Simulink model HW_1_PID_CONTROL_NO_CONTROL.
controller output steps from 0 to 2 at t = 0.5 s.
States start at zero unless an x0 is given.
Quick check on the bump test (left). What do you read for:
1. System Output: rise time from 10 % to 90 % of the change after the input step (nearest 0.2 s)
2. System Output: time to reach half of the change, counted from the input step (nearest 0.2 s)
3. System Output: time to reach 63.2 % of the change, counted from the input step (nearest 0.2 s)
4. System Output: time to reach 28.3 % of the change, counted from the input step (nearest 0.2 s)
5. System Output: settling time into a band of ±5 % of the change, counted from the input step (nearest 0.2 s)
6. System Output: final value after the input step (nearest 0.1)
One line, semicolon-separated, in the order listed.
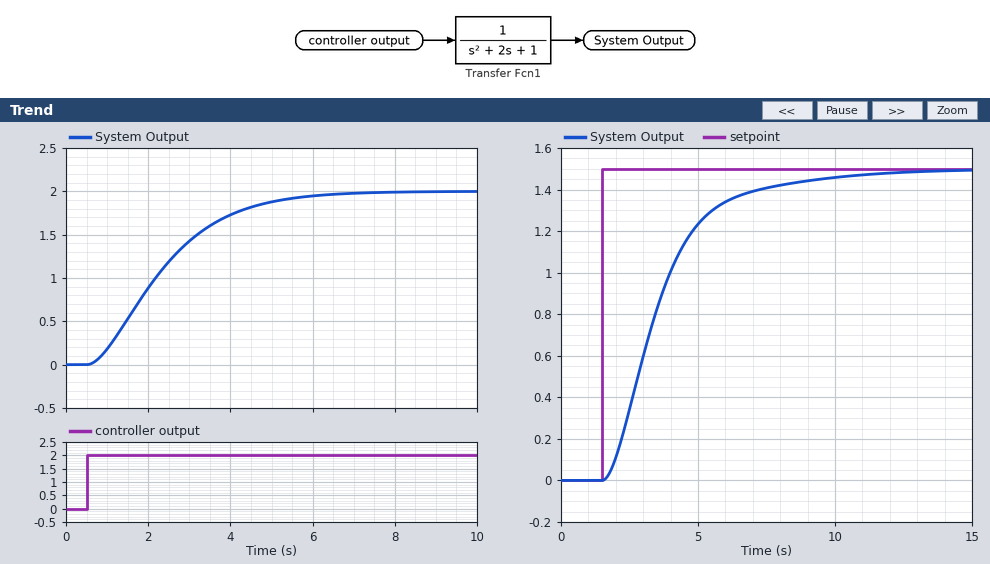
3.4 s; 1.6 s; 2.2 s; 1.0 s; 4.8 s; 2.0
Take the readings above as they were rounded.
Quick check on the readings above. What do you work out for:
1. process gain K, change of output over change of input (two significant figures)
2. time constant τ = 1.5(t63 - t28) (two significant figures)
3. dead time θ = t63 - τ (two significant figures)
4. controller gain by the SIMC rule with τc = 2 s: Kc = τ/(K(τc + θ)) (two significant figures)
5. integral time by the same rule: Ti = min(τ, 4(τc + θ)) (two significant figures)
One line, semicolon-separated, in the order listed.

1.0; 1.8 s; 0.40 s; 0.75; 1.8 s
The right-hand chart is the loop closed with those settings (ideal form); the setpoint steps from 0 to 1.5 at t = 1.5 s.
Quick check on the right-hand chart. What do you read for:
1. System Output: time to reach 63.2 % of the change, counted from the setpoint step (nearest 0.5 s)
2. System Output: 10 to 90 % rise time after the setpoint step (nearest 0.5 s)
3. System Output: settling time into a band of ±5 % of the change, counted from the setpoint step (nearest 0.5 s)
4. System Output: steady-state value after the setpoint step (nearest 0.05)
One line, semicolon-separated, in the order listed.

2.5 s; 4.0 s; 6.5 s; 1.50
